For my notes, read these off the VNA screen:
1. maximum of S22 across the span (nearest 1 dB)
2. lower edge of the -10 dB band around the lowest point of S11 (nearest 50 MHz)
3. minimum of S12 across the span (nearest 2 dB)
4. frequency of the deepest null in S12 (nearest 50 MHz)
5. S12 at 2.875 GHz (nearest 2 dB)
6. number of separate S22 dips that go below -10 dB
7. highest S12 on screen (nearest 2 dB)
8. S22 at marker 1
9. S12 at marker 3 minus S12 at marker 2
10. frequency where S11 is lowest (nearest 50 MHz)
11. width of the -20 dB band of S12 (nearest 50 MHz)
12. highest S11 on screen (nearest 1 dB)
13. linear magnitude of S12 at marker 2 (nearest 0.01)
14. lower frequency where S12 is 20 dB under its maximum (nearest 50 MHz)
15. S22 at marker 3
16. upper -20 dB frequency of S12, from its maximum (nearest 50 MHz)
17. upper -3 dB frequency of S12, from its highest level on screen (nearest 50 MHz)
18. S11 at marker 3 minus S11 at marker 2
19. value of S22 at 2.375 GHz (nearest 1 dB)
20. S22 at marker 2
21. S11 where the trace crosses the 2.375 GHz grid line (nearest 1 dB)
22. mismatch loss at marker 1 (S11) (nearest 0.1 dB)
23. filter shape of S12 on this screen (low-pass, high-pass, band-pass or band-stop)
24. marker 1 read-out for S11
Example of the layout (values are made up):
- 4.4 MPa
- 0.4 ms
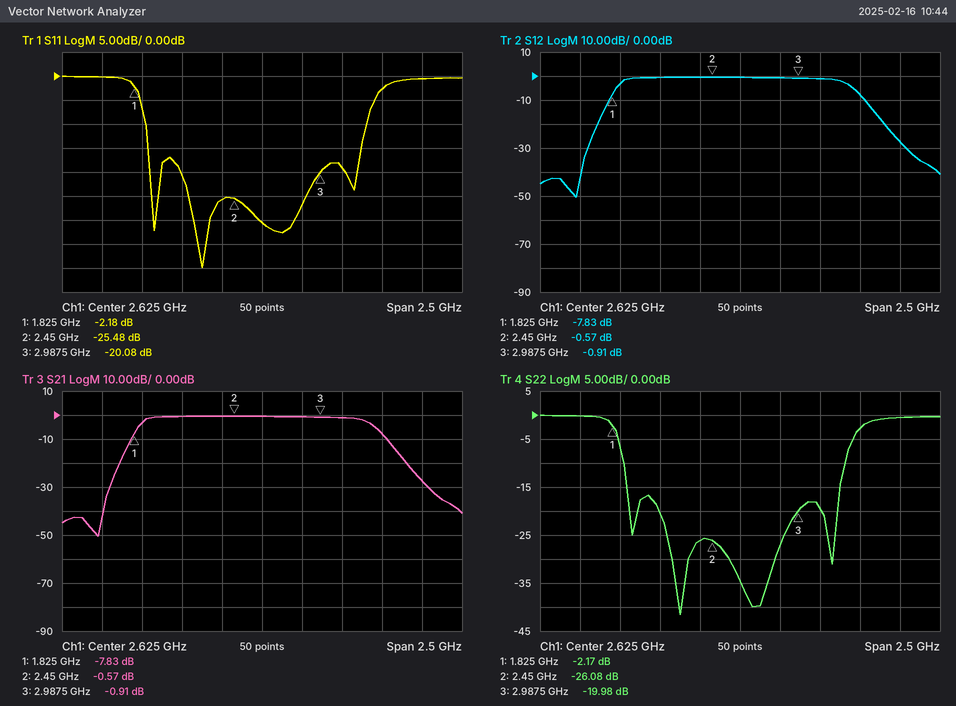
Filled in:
- 0 dB
- 1.90 GHz
- -50 dB
- 1.60 GHz
- 0 dB
- 4
- 0 dB
- -2.17 dB
- -0.34 dB
- 2.25 GHz
- 1.80 GHz
- 0 dB
- 0.94
- 1.75 GHz
- -19.98 dB
- 3.55 GHz
- 3.30 GHz
- 5.40 dB
- -26 dB
- -26.08 dB
- -26 dB
- 4.0 dB
- band-pass
- -2.18 dB
